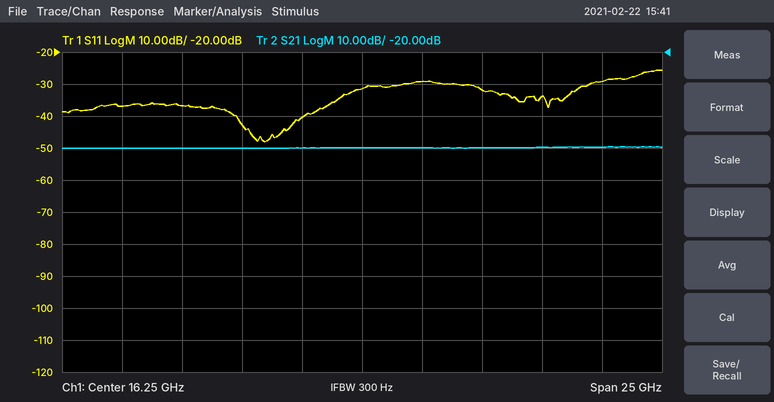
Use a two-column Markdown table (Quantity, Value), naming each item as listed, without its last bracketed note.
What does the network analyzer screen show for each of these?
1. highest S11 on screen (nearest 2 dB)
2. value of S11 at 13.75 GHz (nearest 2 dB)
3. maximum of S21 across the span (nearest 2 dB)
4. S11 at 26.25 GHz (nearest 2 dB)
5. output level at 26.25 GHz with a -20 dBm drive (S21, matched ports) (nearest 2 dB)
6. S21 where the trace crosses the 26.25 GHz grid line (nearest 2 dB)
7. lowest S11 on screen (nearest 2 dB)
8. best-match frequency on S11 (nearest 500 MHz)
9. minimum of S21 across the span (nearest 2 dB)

| Quantity | Value |
|---|---|
| highest S11 on screen | -26 dB |
| value of S11 at 13.75 GHz | -40 dB |
| maximum of S21 across the span | -50 dB |
| S11 at 26.25 GHz | -30 dB |
| output level at 26.25 GHz with a -20 dBm drive (S21, matched ports) | -70 dBm |
| S21 where the trace crosses the 26.25 GHz grid line | -50 dB |
| lowest S11 on screen | -48 dB |
| best-match frequency on S11 | 12.0 GHz |
| minimum of S21 across the span | -50 dB |
